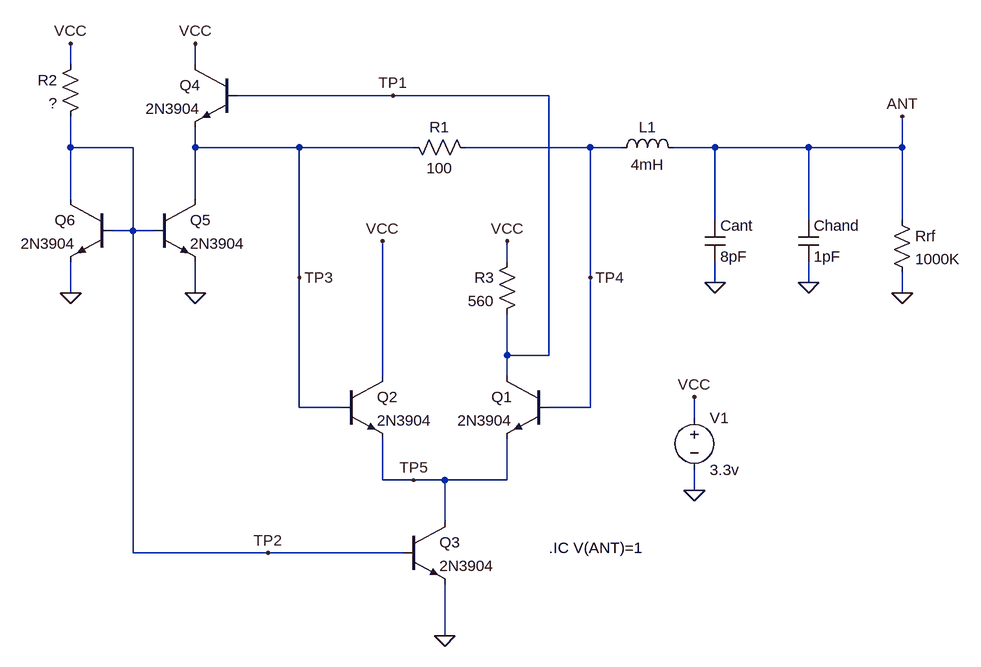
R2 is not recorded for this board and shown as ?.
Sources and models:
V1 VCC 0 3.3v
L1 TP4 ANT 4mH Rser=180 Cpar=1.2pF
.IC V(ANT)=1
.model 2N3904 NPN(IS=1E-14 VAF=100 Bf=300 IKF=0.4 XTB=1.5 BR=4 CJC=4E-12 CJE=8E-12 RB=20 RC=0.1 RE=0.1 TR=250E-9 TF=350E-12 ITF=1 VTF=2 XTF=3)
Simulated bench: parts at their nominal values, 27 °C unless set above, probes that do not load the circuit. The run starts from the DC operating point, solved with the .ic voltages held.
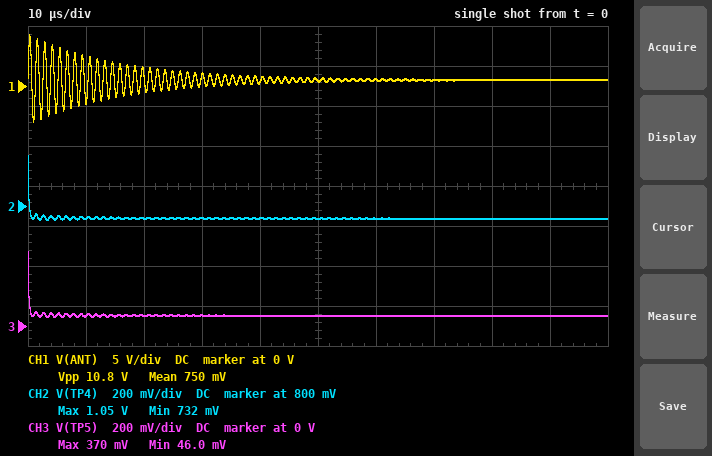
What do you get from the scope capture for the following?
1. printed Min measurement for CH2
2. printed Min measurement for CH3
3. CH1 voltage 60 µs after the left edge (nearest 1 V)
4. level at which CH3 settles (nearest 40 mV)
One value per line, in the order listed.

732 mV
46.0 mV
1 V
40 mV
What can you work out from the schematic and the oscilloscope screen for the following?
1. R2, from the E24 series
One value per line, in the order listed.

240 Ω
